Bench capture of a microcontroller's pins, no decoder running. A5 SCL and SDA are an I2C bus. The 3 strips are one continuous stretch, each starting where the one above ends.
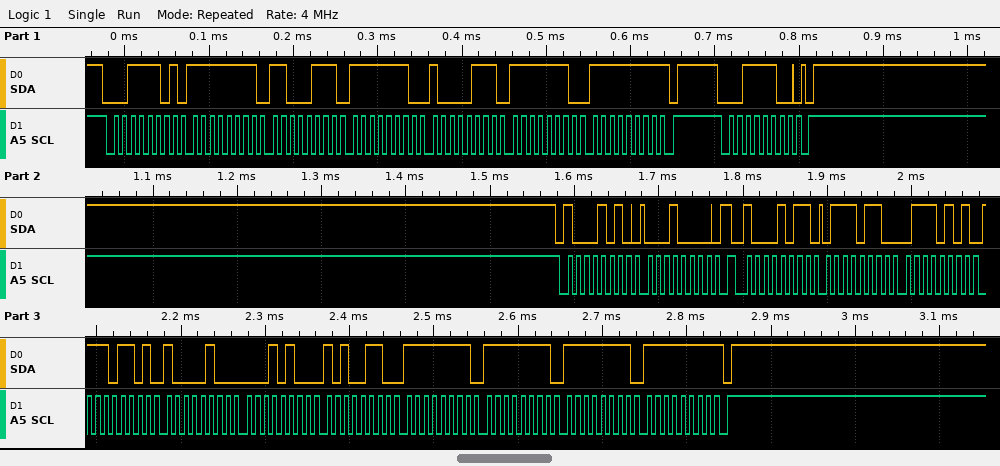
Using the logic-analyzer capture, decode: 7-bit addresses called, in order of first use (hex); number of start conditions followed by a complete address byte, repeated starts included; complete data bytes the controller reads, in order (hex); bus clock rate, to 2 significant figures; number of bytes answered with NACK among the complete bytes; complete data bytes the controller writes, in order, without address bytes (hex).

0x1E 0x45
4
FF C7 FE 87 FE FF 76 75 ED 84 14 A6 FF FF FF FF
100 kHz
2
10
